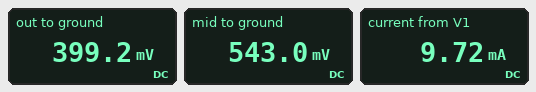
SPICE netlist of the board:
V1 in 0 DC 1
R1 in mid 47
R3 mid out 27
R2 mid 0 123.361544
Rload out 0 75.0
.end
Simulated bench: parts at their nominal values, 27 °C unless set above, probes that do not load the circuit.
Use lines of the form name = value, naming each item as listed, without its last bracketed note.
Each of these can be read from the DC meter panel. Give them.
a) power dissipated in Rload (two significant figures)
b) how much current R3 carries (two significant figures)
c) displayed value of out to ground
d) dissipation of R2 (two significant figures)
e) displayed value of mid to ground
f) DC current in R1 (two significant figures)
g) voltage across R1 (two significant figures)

power dissipated in Rload = 2.1 mW
how much current R3 carries = 5.3 mA
displayed value of out to ground = 399.2 mV
dissipation of R2 = 2.4 mW
displayed value of mid to ground = 543.0 mV
DC current in R1 = 9.7 mA
voltage across R1 = 460 mV
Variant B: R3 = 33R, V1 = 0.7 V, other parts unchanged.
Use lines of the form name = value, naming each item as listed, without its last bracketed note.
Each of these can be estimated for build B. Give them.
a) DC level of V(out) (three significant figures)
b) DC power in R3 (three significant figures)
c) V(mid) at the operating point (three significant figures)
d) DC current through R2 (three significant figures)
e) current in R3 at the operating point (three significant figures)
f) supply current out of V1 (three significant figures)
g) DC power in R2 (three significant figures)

DC level of V(out) = 268 mV
DC power in R3 = 420 µW
V(mid) at the operating point = 385 mV
DC current through R2 = 3.12 mA
current in R3 at the operating point = 3.57 mA
supply current out of V1 = 6.69 mA
DC power in R2 = 1.20 mW
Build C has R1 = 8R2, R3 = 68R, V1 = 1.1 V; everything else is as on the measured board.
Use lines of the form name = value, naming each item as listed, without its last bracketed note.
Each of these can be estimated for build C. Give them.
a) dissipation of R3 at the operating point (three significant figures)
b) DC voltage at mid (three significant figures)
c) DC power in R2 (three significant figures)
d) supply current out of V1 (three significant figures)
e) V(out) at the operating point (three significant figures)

dissipation of R3 at the operating point = 3.19 mW
DC voltage at mid = 979 mV
DC power in R2 = 7.77 mW
supply current out of V1 = 14.8 mA
V(out) at the operating point = 513 mV
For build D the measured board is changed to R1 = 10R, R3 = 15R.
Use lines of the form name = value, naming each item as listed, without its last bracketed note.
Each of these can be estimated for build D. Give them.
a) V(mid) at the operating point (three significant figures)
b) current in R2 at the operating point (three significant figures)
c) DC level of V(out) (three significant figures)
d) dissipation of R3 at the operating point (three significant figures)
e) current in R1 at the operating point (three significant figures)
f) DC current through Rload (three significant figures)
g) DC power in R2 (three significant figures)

V(mid) at the operating point = 839 mV
current in R2 at the operating point = 6.80 mA
DC level of V(out) = 699 mV
dissipation of R3 at the operating point = 1.30 mW
current in R1 at the operating point = 16.1 mA
DC current through Rload = 9.32 mA
DC power in R2 = 5.70 mW
